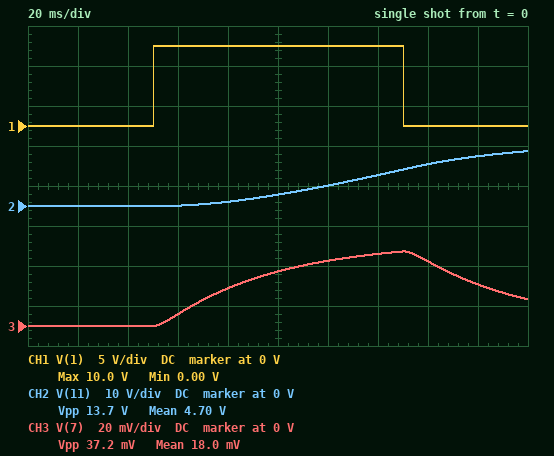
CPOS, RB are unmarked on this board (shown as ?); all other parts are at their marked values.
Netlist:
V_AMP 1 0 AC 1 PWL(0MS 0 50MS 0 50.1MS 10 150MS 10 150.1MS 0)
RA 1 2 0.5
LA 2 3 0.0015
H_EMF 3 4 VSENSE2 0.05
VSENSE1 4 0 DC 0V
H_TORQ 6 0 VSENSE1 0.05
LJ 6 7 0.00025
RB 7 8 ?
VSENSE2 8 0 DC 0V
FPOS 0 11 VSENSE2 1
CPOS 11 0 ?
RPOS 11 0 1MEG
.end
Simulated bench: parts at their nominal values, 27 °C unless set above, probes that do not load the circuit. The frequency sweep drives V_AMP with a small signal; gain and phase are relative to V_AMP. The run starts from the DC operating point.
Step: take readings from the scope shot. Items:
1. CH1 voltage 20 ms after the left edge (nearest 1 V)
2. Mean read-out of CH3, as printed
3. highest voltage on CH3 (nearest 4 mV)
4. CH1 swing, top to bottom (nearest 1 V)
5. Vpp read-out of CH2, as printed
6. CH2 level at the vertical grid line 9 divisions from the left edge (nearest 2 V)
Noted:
0 V
18.0 mV
36 mV
10 V
13.7 V
12 V
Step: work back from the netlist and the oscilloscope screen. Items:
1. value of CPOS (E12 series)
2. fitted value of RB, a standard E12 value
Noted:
1.2 F
220 µΩ
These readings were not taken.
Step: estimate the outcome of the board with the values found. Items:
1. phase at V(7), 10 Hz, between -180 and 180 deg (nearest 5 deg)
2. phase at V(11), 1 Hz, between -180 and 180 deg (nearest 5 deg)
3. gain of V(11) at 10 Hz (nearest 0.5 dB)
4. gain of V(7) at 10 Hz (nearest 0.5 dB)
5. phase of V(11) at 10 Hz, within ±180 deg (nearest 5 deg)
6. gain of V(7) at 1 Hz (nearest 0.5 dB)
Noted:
-80 deg
-105 deg
-21.5 dB
-57.0 dB
-170 deg
-48.0 dB
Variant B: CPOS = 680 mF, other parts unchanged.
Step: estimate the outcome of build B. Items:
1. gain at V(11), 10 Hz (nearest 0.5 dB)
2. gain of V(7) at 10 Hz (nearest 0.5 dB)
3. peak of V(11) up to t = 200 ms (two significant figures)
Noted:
-16.5 dB
-57.0 dB
24 V
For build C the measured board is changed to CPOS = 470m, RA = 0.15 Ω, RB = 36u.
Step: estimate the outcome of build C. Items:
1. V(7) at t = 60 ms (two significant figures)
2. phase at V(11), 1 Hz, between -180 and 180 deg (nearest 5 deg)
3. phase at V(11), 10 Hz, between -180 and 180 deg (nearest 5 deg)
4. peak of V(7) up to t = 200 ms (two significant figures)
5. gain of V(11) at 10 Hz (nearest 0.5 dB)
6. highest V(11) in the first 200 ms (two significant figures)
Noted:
1.7 mV
-95 deg
-155 deg
7.8 mV
-3.5 dB
43 V
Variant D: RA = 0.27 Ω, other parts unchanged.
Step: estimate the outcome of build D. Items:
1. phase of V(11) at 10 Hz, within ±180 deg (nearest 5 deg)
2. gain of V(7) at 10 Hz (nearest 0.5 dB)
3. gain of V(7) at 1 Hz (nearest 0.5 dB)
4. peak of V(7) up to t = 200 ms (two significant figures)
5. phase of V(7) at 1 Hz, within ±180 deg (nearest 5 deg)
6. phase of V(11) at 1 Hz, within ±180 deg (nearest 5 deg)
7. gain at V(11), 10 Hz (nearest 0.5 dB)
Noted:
-165 deg
-52.0 dB
-47.5 dB
43 mV
-10 deg
-100 deg
-16.5 dB
